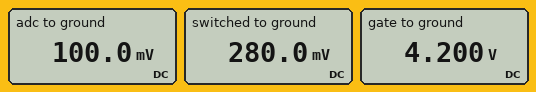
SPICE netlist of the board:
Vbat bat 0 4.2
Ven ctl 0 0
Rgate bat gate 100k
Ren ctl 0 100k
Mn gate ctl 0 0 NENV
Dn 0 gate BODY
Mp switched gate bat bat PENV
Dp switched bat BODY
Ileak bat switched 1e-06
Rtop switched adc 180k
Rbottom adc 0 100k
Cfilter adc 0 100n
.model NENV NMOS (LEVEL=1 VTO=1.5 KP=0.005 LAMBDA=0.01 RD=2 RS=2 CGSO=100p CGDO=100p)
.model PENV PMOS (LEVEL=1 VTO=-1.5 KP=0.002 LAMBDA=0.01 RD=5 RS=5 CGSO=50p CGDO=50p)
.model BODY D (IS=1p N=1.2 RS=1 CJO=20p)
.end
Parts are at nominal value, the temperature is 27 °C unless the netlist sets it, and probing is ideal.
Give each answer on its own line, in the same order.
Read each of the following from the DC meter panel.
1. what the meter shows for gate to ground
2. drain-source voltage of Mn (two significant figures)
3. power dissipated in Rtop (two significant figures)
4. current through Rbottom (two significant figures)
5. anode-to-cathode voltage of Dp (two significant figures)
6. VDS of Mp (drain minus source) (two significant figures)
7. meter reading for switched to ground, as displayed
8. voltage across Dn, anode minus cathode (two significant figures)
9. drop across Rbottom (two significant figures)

4.200 V
4.2 V
180 nW
1.0 µA
-3.9 V
-3.9 V
280.0 mV
-4.2 V
100 mV
